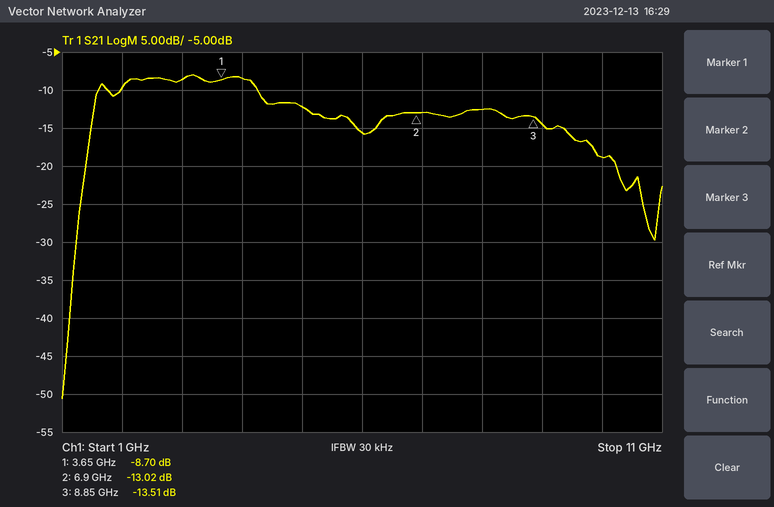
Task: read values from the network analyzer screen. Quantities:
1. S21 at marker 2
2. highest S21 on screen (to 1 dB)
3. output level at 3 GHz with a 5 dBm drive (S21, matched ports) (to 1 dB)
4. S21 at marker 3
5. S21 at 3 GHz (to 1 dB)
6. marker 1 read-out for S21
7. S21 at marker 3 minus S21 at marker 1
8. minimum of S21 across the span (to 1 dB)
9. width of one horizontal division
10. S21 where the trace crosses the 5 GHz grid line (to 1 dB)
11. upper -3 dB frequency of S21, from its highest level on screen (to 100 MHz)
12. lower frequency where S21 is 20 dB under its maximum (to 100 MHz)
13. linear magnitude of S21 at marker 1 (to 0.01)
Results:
-13.02 dB
-8 dB
-4 dBm
-13.51 dB
-9 dB
-8.70 dB
-4.81 dB
-51 dB
1 GHz
-12 dB
4.3 GHz
1.3 GHz
0.37
